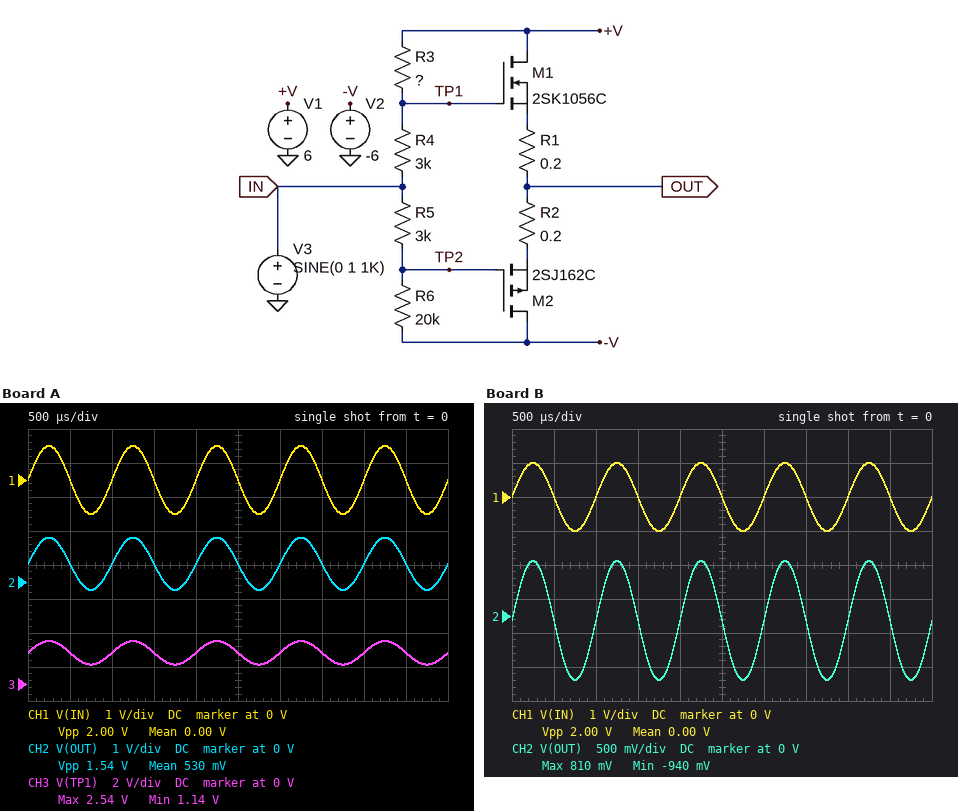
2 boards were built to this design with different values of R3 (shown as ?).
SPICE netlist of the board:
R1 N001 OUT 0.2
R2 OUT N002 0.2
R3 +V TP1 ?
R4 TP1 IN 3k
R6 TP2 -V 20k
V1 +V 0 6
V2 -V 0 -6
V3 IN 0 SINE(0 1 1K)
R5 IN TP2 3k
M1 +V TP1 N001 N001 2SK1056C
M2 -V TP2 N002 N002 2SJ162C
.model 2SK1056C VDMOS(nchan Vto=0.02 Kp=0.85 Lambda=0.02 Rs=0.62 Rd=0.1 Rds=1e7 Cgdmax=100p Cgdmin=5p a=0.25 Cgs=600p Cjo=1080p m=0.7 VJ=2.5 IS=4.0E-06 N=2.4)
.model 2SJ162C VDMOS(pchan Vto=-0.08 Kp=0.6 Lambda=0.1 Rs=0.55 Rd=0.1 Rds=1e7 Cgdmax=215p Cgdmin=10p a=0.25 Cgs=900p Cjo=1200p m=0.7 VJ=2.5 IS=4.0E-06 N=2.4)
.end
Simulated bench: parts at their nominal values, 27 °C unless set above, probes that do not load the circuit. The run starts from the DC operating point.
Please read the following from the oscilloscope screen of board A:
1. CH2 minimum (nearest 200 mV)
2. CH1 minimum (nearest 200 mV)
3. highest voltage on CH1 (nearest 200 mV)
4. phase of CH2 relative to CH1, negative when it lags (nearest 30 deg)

-200 mV
-1.0 V
1.0 V
0 deg
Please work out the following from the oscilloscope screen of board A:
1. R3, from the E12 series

6.8 kΩ
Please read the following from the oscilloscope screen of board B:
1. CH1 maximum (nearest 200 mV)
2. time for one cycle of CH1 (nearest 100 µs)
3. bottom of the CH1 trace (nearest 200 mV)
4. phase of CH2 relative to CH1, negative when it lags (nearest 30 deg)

1.0 V
1.0 ms
-1.0 V
0 deg
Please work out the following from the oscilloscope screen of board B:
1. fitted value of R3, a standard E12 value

27 kΩ
